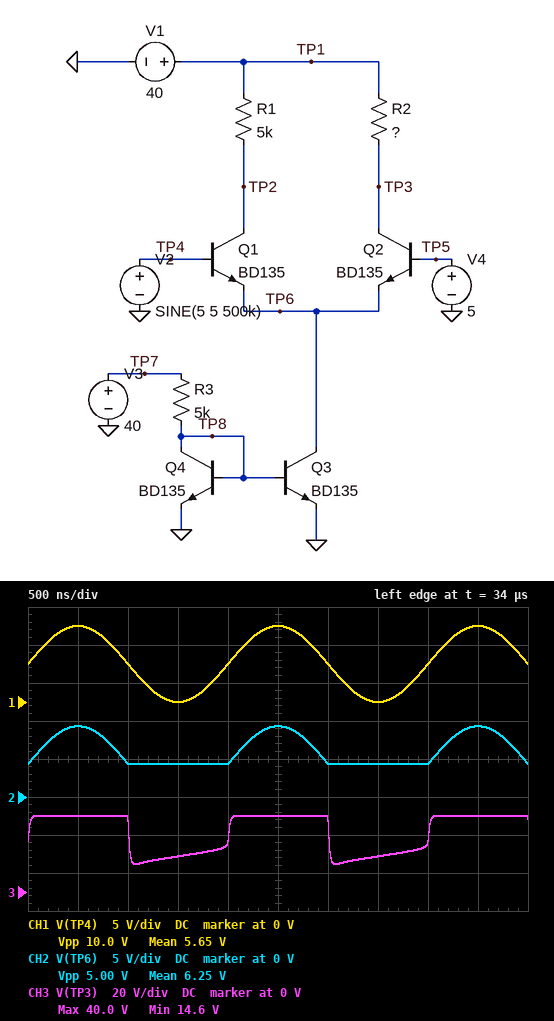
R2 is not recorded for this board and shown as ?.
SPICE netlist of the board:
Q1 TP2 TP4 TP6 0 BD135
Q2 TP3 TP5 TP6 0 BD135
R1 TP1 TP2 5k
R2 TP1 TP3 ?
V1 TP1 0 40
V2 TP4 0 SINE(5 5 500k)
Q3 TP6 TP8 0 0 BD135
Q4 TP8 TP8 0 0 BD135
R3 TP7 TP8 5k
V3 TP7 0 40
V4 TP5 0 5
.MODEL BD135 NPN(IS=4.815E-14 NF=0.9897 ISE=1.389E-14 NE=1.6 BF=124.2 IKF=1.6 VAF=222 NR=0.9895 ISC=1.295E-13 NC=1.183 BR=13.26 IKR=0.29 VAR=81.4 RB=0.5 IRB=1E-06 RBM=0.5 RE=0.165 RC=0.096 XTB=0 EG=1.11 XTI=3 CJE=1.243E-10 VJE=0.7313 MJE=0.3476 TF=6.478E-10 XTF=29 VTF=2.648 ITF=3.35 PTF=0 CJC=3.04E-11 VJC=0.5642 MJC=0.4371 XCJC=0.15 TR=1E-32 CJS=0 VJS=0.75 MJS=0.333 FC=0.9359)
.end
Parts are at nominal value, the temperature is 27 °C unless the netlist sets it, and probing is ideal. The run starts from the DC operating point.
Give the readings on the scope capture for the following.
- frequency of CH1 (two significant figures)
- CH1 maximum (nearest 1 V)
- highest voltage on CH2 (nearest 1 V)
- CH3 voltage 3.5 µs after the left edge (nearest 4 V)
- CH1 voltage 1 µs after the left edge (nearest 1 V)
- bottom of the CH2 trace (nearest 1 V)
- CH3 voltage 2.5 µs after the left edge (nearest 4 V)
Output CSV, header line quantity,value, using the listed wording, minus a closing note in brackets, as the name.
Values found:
quantity,value
frequency of CH1,500 kHz
CH1 maximum,10 V
highest voltage on CH2,9 V
CH3 voltage 3.5 µs after the left edge,20 V
CH1 voltage 1 µs after the left edge,5 V
bottom of the CH2 trace,4 V
CH3 voltage 2.5 µs after the left edge,40 V
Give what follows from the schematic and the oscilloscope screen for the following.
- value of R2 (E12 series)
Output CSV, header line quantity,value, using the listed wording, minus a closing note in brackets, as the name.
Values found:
quantity,value
value of R2,2.7 kΩ
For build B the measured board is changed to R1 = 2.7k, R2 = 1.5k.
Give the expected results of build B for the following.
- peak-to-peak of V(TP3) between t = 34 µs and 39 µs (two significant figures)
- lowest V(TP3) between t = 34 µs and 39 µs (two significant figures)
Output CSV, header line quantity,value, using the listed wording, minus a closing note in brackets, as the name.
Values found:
quantity,value
peak-to-peak of V(TP3) between t = 34 µs and 39 µs,15 V
lowest V(TP3) between t = 34 µs and 39 µs,25 V
